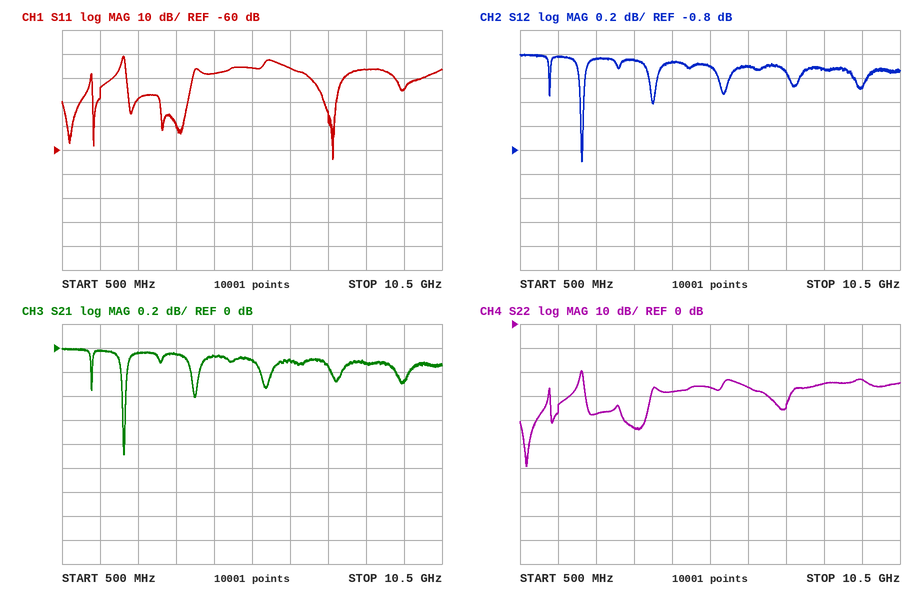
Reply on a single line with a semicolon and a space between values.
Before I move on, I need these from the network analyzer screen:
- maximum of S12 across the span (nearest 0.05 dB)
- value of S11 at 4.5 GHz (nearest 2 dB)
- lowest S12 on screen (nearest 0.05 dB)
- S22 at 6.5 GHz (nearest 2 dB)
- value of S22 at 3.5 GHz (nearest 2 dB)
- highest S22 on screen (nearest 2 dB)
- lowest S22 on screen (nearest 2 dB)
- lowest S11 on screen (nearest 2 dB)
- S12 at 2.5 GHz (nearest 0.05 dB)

0.00 dB; -28 dB; -0.90 dB; -26 dB; -44 dB; -20 dB; -60 dB; -64 dB; -0.05 dB
